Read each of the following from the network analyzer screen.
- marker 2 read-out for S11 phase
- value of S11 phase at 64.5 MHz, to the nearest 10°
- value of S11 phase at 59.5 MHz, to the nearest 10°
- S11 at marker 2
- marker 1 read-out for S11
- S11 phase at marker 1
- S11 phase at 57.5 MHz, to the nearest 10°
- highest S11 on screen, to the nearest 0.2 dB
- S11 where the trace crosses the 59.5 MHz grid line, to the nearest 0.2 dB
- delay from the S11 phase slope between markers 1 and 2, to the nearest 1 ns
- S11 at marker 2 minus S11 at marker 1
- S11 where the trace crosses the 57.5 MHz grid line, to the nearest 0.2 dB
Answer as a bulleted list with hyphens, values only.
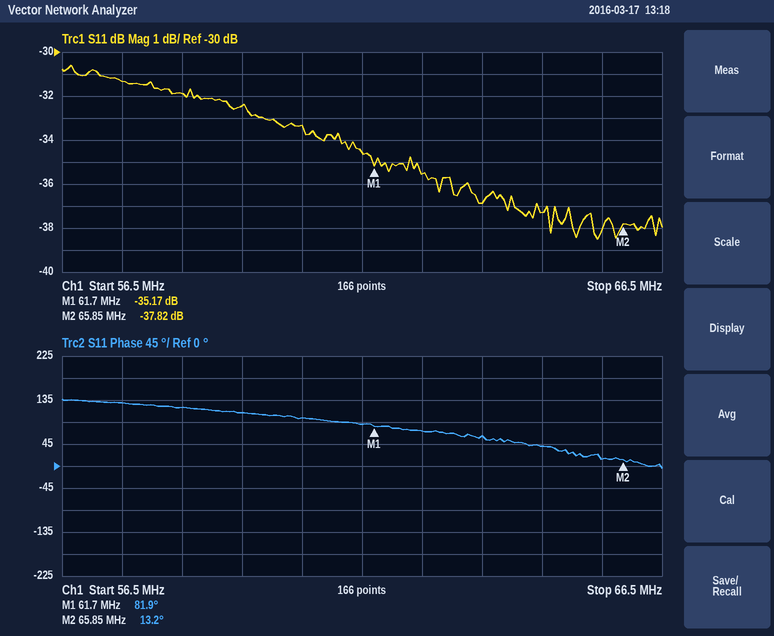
- 13.2°
- 40°
- 110°
- -37.82 dB
- -35.17 dB
- 81.9°
- 130°
- -30.6 dB
- -32.4 dB
- 46 ns
- -2.65 dB
- -31.4 dB
